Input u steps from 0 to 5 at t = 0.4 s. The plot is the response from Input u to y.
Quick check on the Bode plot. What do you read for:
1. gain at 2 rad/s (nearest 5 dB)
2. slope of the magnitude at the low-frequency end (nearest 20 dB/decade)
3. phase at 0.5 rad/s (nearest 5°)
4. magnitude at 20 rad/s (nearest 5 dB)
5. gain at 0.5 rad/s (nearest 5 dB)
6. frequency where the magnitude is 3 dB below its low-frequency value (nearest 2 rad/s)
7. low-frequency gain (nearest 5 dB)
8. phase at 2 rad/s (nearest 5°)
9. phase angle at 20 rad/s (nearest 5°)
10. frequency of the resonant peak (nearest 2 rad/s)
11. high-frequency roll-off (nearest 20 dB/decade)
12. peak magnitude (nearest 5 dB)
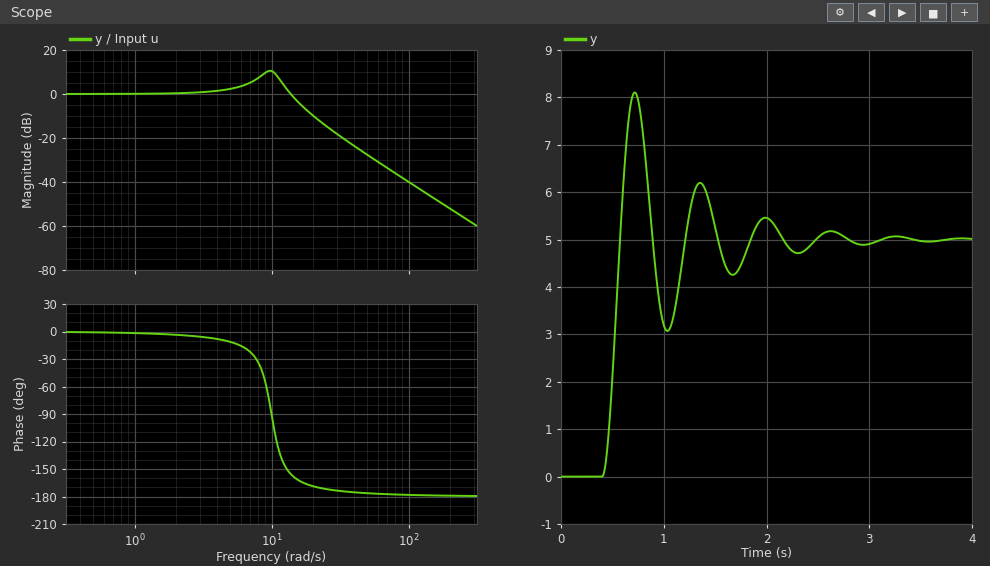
0 dB
0 dB/decade
0°
-10 dB
0 dB
16 rad/s
0 dB
-5°
-170°
10 rad/s
-40 dB/decade
10 dB
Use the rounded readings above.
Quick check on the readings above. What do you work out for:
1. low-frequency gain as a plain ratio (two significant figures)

1.0
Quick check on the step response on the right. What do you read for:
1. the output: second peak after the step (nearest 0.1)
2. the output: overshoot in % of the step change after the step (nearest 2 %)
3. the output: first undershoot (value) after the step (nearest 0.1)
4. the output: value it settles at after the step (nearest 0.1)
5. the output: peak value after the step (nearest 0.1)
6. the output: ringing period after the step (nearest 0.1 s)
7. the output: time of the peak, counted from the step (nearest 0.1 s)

6.2
62 %
3.1
5.0
8.1
0.6 s
0.3 s
